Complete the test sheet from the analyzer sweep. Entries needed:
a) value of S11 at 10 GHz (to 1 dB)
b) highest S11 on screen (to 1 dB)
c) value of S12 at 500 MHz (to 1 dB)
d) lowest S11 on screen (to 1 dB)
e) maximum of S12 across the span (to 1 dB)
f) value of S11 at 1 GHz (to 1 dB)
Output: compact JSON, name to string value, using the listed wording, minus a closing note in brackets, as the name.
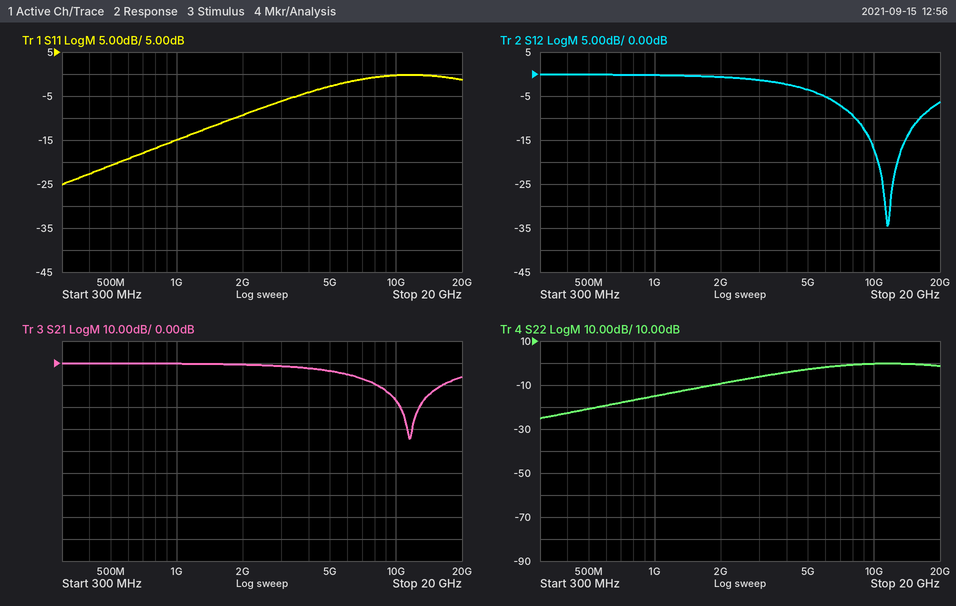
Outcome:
{"value of S11 at 10 GHz": "0 dB", "highest S11 on screen": "0 dB", "value of S12 at 500 MHz": "0 dB", "lowest S11 on screen": "-25 dB", "maximum of S12 across the span": "0 dB", "value of S11 at 1 GHz": "-15 dB"}
